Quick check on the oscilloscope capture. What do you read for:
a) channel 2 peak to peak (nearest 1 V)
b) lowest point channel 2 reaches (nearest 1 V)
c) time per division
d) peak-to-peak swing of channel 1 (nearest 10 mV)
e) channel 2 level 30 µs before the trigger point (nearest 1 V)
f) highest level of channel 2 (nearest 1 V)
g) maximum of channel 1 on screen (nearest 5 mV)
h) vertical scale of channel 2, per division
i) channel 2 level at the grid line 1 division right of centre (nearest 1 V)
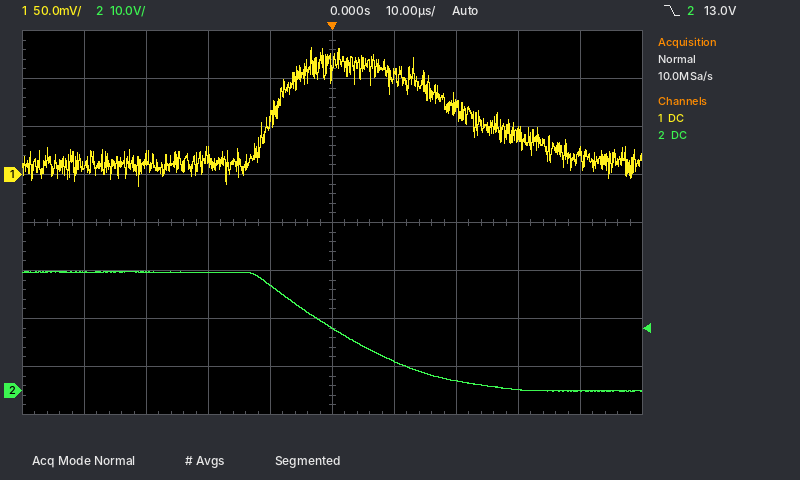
25 V
0 V
10 µs
140 mV
25 V
25 V
130 mV
10 V
6 V
